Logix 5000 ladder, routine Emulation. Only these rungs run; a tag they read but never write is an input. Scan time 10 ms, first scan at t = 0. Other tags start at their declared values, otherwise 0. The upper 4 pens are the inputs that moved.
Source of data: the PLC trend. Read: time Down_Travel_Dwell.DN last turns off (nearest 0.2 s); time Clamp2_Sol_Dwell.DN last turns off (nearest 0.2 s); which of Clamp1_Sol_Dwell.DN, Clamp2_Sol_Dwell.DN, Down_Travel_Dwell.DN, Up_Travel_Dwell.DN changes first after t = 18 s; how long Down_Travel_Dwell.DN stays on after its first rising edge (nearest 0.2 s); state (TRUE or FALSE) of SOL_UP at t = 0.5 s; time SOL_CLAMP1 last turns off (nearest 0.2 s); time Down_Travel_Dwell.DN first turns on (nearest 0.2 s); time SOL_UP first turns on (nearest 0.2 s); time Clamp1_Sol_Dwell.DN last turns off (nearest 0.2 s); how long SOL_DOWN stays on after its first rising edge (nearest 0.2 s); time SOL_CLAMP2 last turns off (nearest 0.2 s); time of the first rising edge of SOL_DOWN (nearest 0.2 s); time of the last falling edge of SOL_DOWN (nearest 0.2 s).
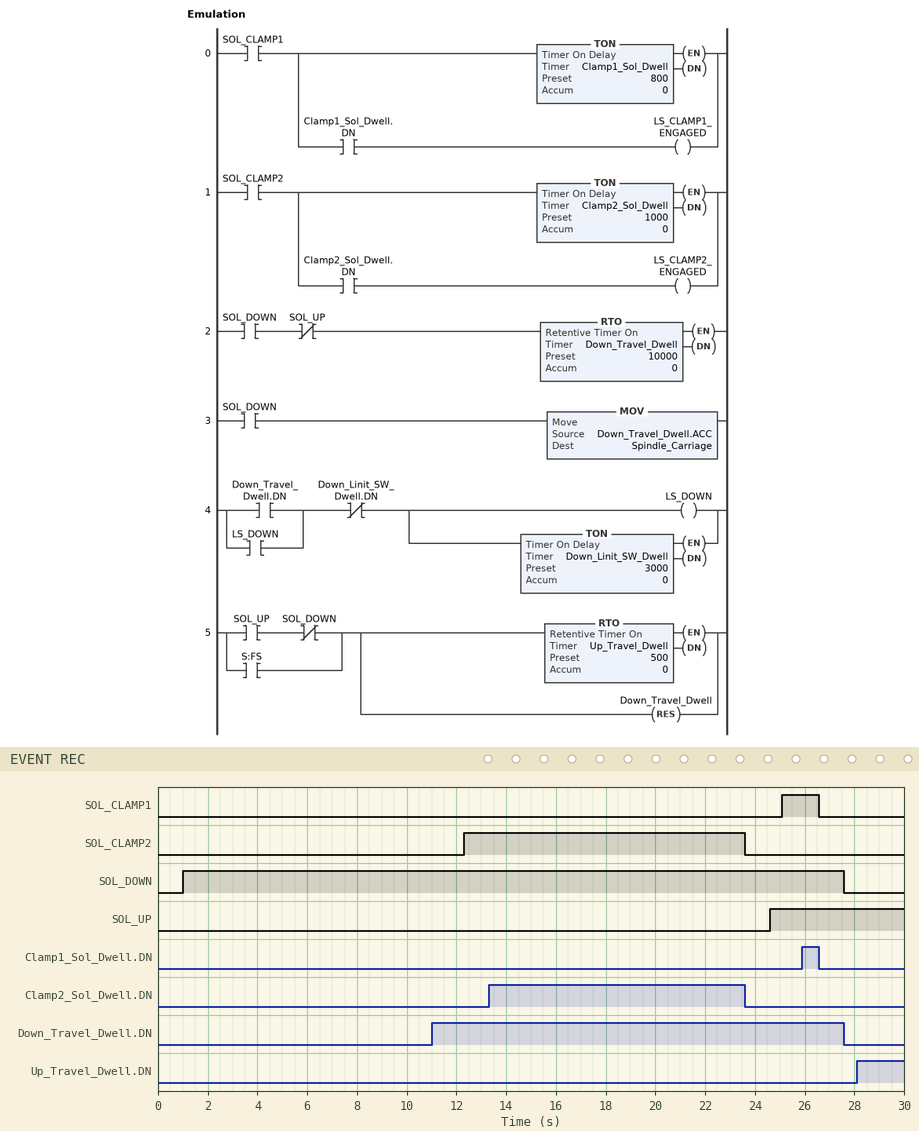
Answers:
27.6 s
23.6 s
Clamp2_Sol_Dwell.DN
16.6 s
FALSE
26.6 s
11.0 s
24.6 s
26.6 s
26.6 s
23.6 s
1.0 s
27.6 s
